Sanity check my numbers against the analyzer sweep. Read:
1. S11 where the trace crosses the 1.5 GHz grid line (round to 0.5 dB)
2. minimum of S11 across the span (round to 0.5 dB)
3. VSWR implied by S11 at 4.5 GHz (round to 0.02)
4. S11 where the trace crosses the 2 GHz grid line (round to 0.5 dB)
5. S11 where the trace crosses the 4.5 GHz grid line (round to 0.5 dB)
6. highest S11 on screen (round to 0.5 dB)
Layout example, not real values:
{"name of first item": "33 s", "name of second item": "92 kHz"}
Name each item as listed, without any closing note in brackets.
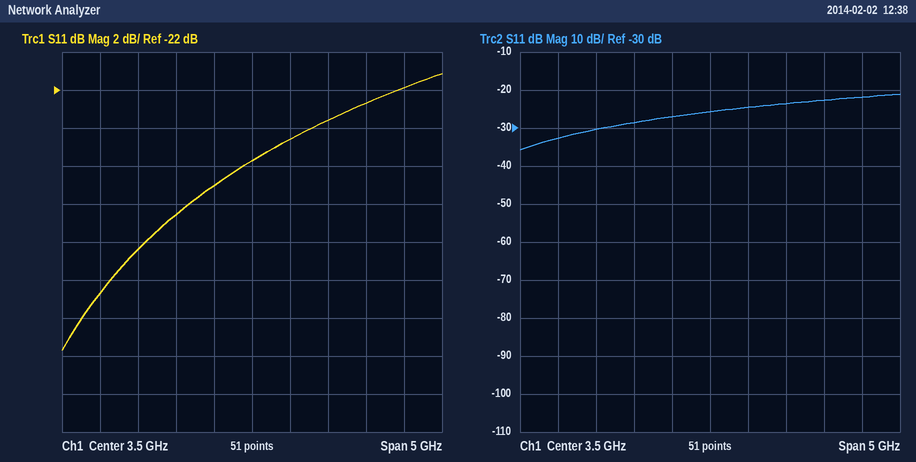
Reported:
{"S11 where the trace crosses the 1.5 GHz grid line": "-32.5 dB", "minimum of S11 across the span": "-35.5 dB", "VSWR implied by S11 at 4.5 GHz": "1.14", "S11 where the trace crosses the 2 GHz grid line": "-30.5 dB", "S11 where the trace crosses the 4.5 GHz grid line": "-23.5 dB", "highest S11 on screen": "-21.0 dB"}
